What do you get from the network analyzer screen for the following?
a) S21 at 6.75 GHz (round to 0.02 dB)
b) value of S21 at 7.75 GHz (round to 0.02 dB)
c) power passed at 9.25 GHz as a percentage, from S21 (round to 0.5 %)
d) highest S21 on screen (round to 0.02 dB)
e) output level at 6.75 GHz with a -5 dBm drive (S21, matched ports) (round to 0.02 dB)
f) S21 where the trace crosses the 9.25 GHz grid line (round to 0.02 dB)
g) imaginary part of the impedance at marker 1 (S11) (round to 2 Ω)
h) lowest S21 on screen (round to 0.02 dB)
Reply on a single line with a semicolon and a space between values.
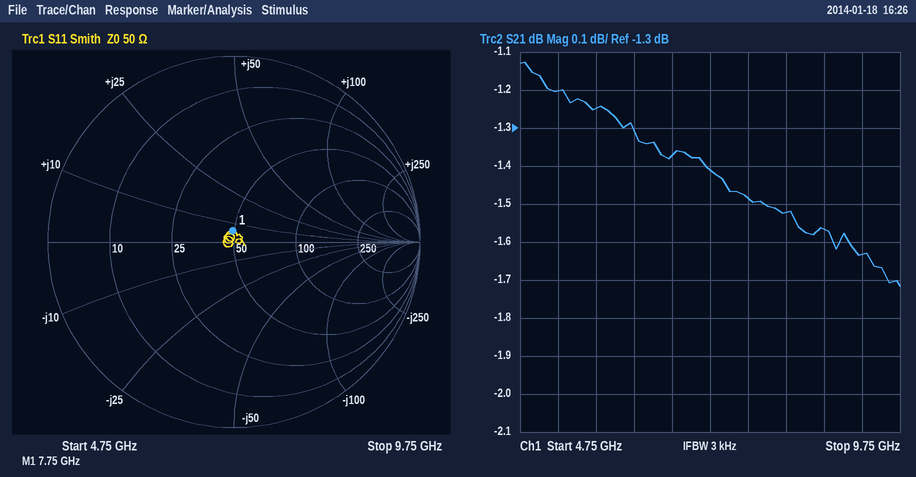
-1.38 dB; -1.48 dB; 68.5 %; -1.12 dB; -6.38 dBm; -1.64 dB; +6 Ω; -1.72 dB
